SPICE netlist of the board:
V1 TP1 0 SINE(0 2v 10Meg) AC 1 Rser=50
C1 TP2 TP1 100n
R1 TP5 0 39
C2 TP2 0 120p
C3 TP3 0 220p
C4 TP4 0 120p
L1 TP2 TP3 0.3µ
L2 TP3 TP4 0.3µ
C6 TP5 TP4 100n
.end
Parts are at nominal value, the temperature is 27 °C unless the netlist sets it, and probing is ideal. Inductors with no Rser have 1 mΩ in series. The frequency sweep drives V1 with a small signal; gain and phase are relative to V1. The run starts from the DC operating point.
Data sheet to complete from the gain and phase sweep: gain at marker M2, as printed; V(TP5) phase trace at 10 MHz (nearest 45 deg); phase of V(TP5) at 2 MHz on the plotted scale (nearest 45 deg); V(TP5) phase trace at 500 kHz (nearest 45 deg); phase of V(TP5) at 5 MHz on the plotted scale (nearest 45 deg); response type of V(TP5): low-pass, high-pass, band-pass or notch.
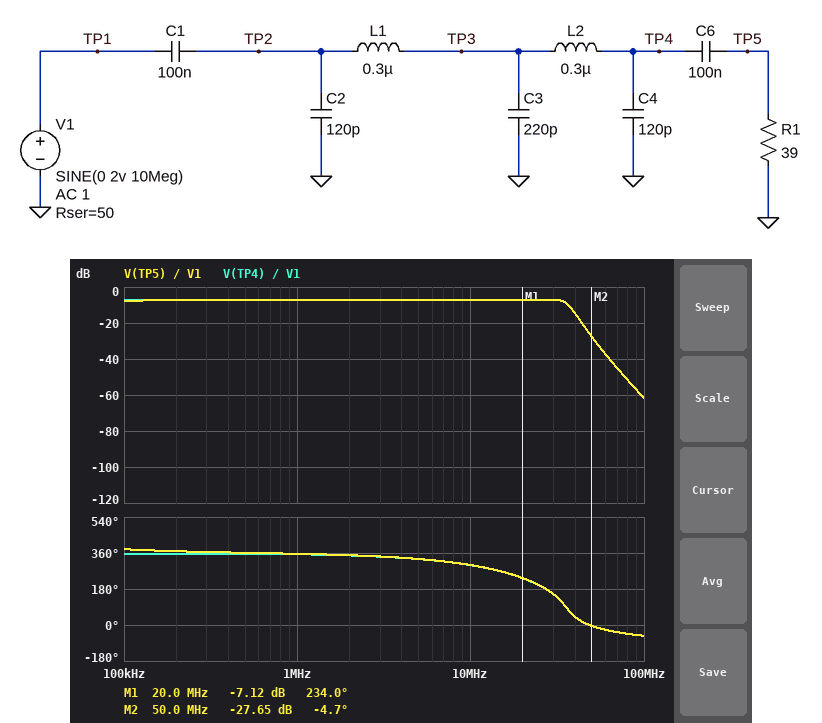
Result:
-27.65 dB
315 deg
360 deg
360 deg
315 deg
low-pass
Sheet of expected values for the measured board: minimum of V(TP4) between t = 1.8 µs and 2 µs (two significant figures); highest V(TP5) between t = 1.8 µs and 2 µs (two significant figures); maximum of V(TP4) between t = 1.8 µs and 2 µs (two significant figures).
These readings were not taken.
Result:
-870 mV
870 mV
870 mV
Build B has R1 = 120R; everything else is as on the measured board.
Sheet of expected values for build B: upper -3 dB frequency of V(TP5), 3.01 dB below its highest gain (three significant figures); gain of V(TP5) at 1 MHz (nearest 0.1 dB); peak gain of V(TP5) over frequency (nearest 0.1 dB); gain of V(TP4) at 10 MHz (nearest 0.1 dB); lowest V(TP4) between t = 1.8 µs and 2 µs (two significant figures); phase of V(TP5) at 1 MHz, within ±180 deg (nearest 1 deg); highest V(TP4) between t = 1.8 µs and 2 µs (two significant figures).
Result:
38.4 MHz
-3.1 dB
-2.2 dB
-4.0 dB
-1.3 V
-6 deg
1.3 V
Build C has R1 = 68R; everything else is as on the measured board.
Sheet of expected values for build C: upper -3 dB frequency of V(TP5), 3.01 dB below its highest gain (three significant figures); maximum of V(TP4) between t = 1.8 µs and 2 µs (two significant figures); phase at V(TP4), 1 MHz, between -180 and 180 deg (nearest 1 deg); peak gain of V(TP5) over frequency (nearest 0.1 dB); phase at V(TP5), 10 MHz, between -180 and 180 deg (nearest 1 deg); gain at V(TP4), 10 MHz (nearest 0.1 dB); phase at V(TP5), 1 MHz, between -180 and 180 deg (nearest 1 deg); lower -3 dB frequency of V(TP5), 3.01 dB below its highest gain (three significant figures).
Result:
37.9 MHz
1.1 V
-6 deg
-4.7 dB
-62 deg
-5.3 dB
-5 deg
27.5 kHz
